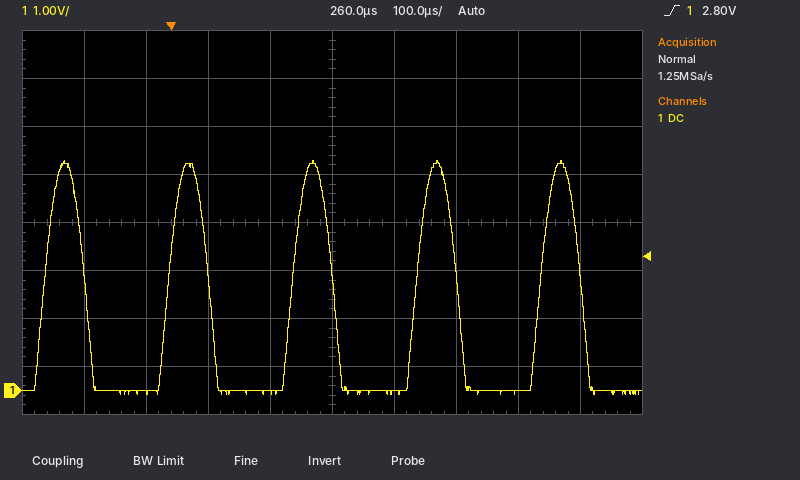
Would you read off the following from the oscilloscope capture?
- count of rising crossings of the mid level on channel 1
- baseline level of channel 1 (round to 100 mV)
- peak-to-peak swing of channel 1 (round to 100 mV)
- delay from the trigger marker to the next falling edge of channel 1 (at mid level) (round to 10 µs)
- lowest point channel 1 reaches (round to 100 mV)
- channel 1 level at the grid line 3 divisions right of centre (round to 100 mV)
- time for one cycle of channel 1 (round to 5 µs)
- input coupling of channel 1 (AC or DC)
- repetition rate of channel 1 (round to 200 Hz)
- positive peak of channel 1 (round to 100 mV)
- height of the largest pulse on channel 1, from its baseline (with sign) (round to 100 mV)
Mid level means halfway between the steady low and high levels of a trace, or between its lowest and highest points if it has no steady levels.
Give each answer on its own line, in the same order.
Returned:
5
0.0 V
4.9 V
60 µs
-100 mV
0.0 V
200 µs
DC
5.0 kHz
4.8 V
+4.8 V
